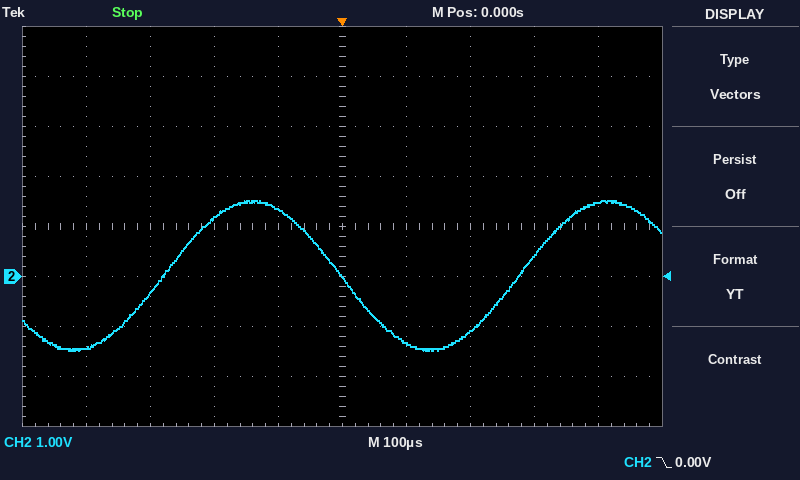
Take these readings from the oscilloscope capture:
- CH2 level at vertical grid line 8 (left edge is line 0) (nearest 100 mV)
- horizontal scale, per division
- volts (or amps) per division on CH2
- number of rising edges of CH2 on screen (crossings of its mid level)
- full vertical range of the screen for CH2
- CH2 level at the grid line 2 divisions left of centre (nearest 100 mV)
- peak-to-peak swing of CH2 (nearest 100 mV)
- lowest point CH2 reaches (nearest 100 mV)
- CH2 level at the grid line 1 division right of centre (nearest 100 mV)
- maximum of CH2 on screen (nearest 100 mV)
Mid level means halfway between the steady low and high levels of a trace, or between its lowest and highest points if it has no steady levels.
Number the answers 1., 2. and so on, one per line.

1. 400 mV
2. 100 µs
3. 1 V
4. 2
5. 8 V
6. 1.2 V
7. 3.0 V
8. -1.5 V
9. -1.3 V
10. 1.5 V
